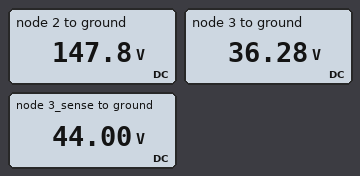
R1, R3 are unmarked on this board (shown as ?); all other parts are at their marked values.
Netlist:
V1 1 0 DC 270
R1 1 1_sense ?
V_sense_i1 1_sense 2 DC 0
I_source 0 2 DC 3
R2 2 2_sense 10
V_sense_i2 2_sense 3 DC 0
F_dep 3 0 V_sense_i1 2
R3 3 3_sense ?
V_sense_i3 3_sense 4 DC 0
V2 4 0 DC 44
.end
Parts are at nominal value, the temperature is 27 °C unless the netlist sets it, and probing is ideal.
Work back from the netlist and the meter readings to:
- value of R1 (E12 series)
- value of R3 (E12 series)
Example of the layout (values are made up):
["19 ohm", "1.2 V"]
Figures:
["15 Ω", "1.5 Ω"]
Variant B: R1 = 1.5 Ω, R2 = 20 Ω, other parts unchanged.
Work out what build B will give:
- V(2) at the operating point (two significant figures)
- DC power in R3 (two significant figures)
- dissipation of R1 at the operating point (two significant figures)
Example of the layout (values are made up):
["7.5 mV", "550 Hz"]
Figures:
["260 V", "39 W", "98 W"]
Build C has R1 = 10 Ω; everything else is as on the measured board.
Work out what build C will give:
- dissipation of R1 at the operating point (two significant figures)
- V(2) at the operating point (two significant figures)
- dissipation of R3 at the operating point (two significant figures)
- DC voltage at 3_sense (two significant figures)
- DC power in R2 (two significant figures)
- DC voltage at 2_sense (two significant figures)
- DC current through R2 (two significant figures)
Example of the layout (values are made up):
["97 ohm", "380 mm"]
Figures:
["1.1 kW", "170 V", "81 W", "44 V", "1.8 kW", "33 V", "13 A"]
